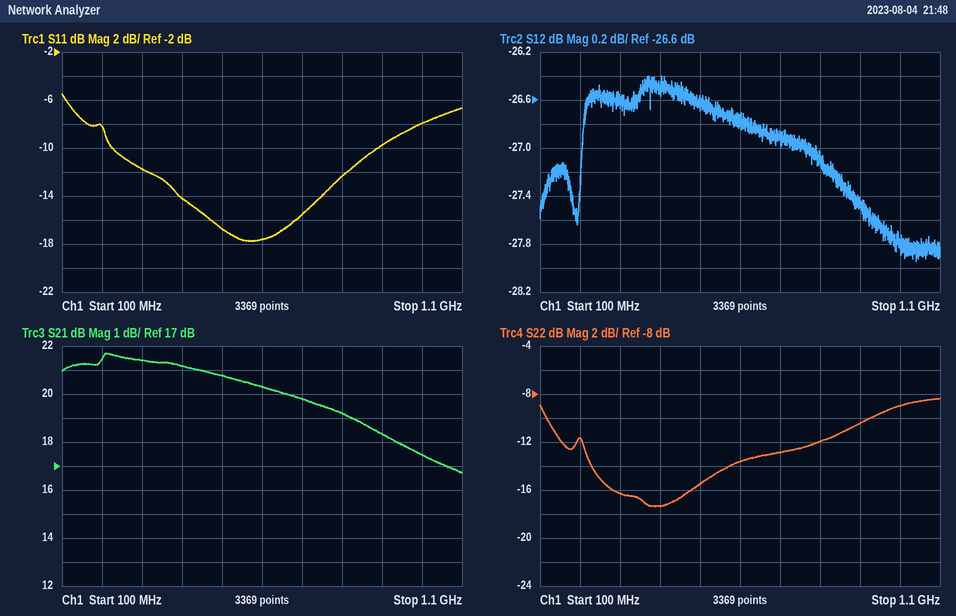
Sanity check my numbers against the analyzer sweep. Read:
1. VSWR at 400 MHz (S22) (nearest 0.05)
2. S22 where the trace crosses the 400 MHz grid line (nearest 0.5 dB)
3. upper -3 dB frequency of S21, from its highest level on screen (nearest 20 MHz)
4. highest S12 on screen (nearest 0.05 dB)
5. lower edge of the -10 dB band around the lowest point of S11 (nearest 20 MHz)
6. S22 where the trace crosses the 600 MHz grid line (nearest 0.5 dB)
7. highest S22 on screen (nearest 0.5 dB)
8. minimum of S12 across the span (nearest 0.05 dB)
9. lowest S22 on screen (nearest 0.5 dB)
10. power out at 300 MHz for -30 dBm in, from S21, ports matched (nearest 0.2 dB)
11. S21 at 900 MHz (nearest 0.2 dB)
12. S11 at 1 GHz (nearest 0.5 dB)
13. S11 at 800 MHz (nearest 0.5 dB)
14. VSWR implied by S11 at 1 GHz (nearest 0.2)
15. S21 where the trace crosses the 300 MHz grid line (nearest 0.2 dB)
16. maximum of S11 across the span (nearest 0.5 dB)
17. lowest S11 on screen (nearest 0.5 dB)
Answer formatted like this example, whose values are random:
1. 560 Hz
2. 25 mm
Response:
1. 1.30
2. -17.5 dB
3. 860 MHz
4. -26.40 dB
5. 220 MHz
6. -13.5 dB
7. -8.5 dB
8. -27.95 dB
9. -17.5 dB
10. -8.6 dBm
11. 18.4 dB
12. -8.0 dB
13. -12.5 dB
14. 2.4
15. 21.4 dB
16. -5.5 dB
17. -18.0 dB
